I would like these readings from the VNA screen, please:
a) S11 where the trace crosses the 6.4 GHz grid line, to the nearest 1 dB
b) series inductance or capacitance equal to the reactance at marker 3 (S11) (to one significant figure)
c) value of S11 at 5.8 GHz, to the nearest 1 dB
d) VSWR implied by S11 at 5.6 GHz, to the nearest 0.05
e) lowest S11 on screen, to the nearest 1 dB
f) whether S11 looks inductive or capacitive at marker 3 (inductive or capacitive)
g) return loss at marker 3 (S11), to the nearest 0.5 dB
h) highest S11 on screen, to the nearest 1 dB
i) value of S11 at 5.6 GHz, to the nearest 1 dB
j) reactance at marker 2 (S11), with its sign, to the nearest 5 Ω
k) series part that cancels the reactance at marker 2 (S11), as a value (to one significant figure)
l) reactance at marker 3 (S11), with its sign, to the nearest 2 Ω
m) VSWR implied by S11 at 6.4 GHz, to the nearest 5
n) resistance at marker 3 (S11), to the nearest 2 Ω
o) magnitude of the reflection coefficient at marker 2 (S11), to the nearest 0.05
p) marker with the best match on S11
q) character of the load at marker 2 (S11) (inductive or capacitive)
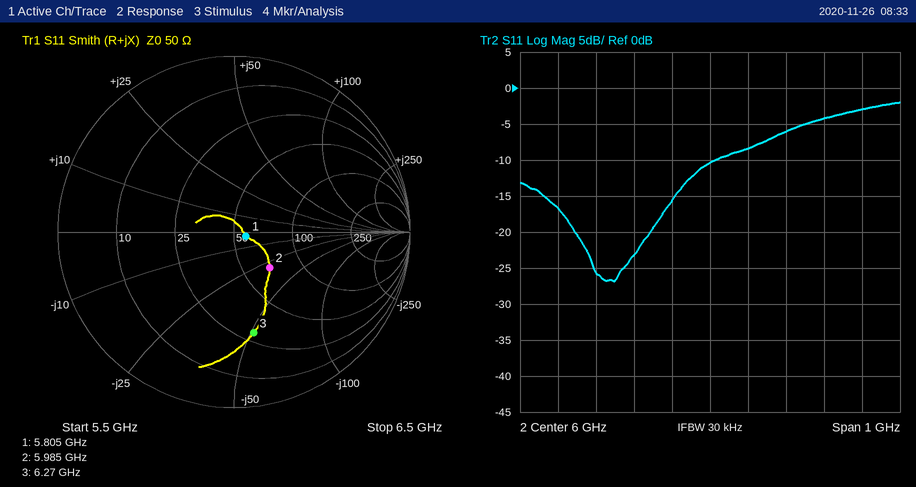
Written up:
-3 dB
500 fF
-23 dB
1.35
-27 dB
capacitive
4.5 dB
-2 dB
-17 dB
-30 Ω
800 pH
-52 Ω
5
30 Ω
0.30
marker 1
capacitive
